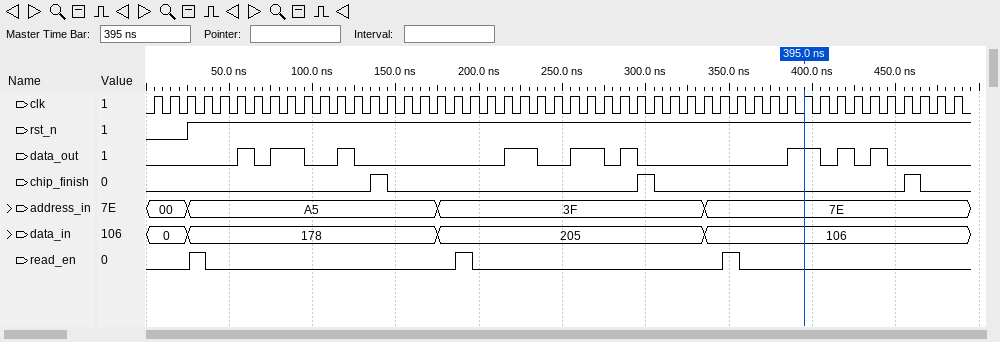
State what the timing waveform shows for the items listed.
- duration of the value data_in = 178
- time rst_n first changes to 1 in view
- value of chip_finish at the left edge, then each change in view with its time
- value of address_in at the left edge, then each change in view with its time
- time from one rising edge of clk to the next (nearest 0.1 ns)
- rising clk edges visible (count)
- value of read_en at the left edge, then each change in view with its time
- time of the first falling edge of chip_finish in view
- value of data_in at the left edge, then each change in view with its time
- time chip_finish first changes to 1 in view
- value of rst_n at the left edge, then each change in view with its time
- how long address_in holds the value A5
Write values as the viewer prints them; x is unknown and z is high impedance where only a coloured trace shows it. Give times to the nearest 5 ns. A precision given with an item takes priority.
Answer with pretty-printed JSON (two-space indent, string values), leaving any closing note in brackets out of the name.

{
  "duration of the value data_in = 178": "150 ns",
  "time rst_n first changes to 1 in view": "25 ns",
  "value of chip_finish at the left edge, then each change in view with its time": "0, 1 at 135 ns, 0 at 145 ns, 1 at 295 ns, 0 at 305 ns, 1 at 455 ns, 0 at 465 ns",
  "value of address_in at the left edge, then each change in view with its time": "00, A5 at 25 ns, 3F at 175 ns, 7E at 335 ns",
  "time from one rising edge of clk to the next": "10 ns",
  "rising clk edges visible": "49",
  "value of read_en at the left edge, then each change in view with its time": "0, 1 at 25 ns, 0 at 35 ns, 1 at 185 ns, 0 at 195 ns, 1 at 345 ns, 0 at 355 ns",
  "time of the first falling edge of chip_finish in view": "145 ns",
  "value of data_in at the left edge, then each change in view with its time": "0, 178 at 25 ns, 205 at 175 ns, 106 at 335 ns",
  "time chip_finish first changes to 1 in view": "135 ns",
  "value of rst_n at the left edge, then each change in view with its time": "0, 1 at 25 ns",
  "how long address_in holds the value A5": "150 ns"
}
